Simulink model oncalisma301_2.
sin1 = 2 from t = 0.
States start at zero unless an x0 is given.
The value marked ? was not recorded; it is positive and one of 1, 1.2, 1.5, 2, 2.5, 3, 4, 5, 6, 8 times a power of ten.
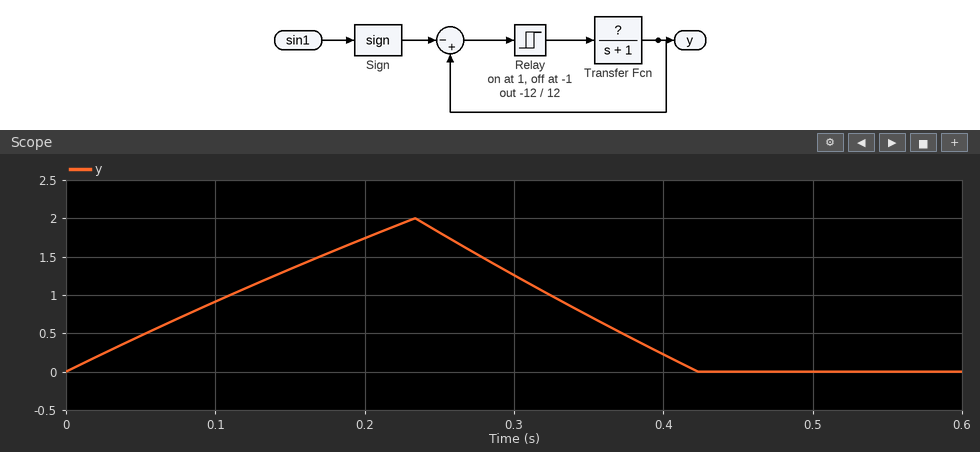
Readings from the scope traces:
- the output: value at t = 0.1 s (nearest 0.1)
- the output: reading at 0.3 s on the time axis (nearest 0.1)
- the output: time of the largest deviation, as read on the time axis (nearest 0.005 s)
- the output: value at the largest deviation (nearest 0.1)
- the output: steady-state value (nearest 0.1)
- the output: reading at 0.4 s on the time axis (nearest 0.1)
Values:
0.9
1.3
0.235 s
2.0
0.0
0.2
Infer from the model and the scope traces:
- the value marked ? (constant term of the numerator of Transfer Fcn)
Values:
0.8
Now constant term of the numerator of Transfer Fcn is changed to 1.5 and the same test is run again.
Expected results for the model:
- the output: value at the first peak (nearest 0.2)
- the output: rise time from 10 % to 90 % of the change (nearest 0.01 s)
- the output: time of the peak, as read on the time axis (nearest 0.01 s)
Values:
2.0
0.04 s
0.12 s
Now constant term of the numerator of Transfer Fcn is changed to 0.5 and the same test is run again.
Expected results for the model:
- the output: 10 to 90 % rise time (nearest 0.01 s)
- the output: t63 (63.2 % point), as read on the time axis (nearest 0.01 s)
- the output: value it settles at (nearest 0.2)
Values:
0.32 s
0.24 s
2.0
